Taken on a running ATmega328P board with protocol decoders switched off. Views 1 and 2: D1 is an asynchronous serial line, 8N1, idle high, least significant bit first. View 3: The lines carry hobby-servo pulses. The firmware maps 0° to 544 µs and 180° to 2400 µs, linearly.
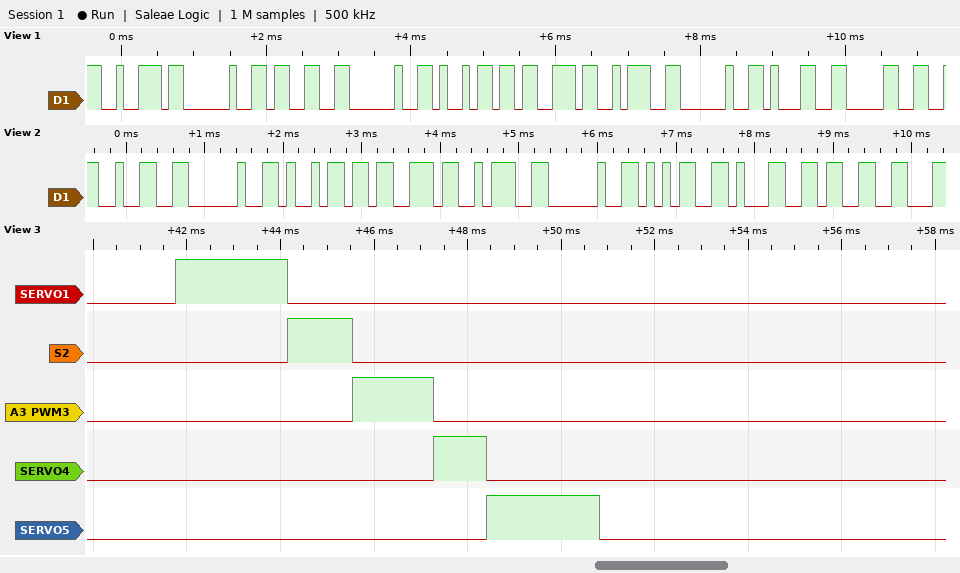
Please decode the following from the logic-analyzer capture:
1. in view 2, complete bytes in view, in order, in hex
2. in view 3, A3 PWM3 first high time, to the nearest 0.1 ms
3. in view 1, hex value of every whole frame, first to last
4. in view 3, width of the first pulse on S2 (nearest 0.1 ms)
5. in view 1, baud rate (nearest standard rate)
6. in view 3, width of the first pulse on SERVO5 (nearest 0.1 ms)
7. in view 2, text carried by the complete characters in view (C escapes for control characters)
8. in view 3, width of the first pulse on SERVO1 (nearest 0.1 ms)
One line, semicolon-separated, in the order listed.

32 20 69 73 3A 20 35 31 33; 1.7 ms; 72 20 33 20 69 73 3A 20 31 30; 1.4 ms; 9600 baud; 2.4 ms; "2 is: 513"; 2.4 ms
